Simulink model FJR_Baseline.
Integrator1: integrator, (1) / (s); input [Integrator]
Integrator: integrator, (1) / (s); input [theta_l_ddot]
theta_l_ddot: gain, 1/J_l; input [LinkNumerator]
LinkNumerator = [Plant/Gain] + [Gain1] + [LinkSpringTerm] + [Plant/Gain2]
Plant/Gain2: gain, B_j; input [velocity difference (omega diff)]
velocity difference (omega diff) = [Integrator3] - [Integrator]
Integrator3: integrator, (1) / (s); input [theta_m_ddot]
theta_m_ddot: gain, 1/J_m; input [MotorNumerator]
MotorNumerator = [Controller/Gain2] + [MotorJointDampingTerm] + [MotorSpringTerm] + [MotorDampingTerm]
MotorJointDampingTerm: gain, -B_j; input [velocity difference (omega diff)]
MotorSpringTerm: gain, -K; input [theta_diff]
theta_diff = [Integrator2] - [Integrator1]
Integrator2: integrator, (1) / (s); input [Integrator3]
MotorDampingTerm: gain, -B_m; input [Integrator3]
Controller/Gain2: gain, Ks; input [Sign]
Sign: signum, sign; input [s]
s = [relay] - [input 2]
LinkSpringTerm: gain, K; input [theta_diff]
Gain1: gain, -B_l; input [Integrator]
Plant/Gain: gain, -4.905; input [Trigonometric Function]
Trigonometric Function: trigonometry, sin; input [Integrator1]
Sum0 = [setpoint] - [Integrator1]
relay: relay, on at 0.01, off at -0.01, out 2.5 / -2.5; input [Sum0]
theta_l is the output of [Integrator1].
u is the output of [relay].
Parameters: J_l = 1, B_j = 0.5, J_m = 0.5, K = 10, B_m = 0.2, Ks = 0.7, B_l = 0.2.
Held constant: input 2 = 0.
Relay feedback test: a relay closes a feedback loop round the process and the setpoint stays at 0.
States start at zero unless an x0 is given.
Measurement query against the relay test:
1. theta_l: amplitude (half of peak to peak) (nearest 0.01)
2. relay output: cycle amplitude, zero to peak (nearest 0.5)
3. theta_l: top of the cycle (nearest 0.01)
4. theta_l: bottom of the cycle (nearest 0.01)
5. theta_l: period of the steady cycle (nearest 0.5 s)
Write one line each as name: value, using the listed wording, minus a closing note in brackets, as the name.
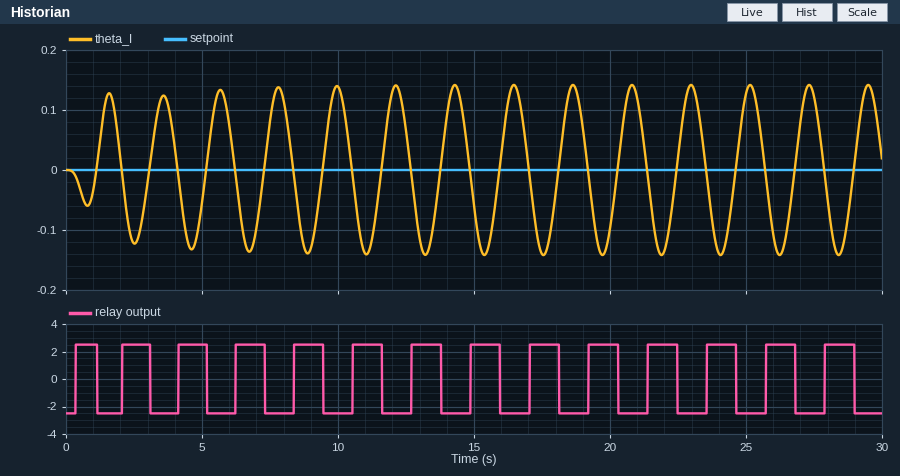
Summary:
theta_l: amplitude (half of peak to peak): 0.14
relay output: cycle amplitude, zero to peak: 2.5
theta_l: top of the cycle: 0.14
theta_l: bottom of the cycle: -0.14
theta_l: period of the steady cycle: 2.0 s
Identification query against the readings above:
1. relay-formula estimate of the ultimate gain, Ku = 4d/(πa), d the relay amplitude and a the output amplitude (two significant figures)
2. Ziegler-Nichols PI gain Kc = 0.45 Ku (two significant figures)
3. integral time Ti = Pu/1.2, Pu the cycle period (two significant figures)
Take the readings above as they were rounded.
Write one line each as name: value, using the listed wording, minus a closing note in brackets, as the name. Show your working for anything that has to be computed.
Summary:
relay-formula estimate of the ultimate gain, Ku = 4d/(πa), d the relay amplitude and a the output amplitude: 4 × 2.5 / (π × 0.14) = 23
Ziegler-Nichols PI gain Kc = 0.45 Ku: 0.45 × 23 = 10
integral time Ti = Pu/1.2, Pu the cycle period: 2 / 1.2 = 1.7 s
